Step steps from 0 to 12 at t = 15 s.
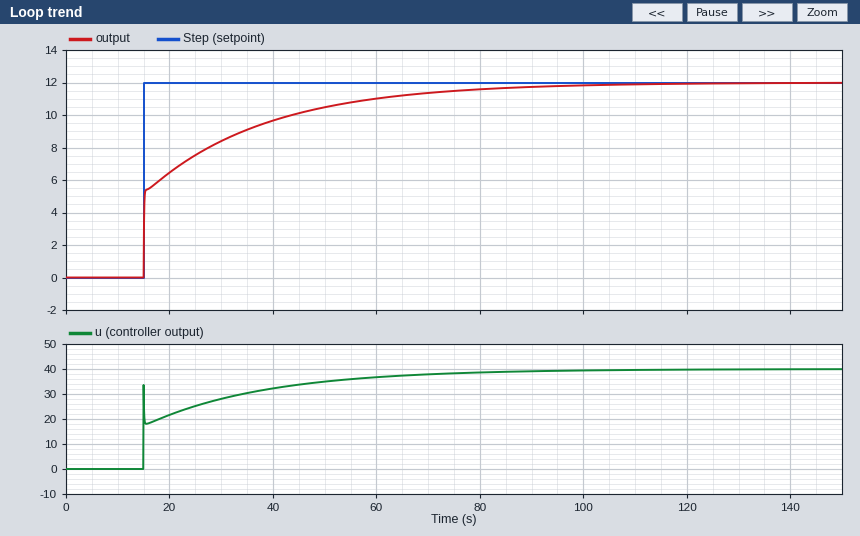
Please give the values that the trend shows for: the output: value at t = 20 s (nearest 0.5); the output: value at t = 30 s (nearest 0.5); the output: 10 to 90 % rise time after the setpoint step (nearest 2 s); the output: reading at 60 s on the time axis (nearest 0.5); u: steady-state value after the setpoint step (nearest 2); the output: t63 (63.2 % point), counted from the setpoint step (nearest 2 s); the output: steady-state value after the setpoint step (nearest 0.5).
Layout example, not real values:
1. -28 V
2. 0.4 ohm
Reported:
1. 6.5
2. 8.5
3. 40 s
4. 11.0
5. 40
6. 10 s
7. 12.0
